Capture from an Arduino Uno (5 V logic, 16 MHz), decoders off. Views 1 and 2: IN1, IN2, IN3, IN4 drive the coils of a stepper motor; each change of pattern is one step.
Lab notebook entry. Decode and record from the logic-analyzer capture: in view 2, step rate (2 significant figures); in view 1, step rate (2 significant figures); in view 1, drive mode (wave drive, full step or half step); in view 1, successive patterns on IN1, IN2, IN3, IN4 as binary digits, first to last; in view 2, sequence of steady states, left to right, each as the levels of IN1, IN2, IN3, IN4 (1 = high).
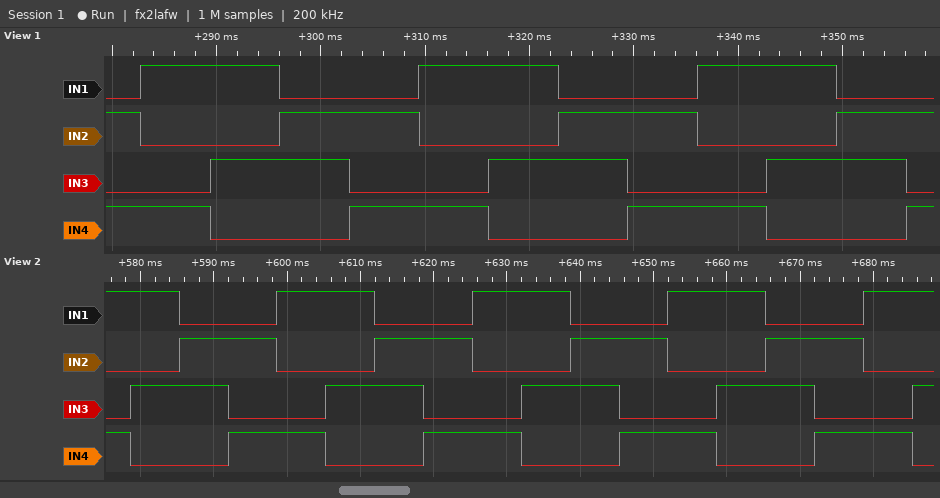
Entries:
150 steps/s
150 steps/s
full step
0101 1001 1010 0110 0101 1001 1010 0110 0101 1001 1010 0110 0101
1001 1010 0110 0101 1001 1010 0110 0101 1001 1010 0110 0101 1001 1010 0110 0101 1001 1010
